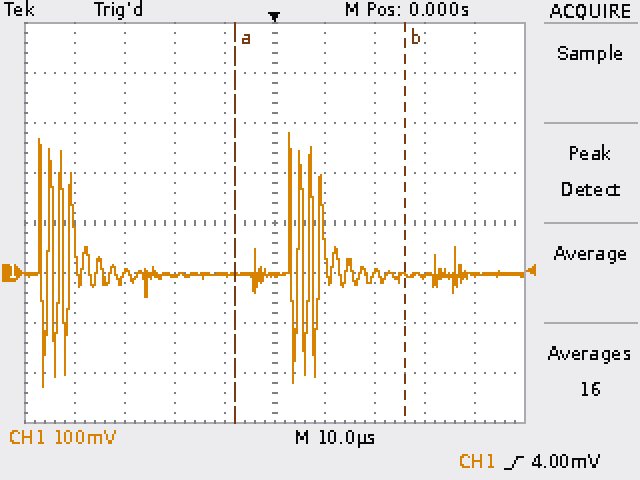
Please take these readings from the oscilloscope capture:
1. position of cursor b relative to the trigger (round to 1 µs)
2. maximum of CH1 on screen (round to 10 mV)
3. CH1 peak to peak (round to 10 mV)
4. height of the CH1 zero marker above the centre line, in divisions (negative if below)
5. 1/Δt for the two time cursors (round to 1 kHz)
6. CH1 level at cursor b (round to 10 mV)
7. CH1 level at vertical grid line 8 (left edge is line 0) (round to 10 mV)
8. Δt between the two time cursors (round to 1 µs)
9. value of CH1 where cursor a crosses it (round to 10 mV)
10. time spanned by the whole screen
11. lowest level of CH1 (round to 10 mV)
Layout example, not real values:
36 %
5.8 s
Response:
+26 µs
280 mV
510 mV
-1.0 div
29 kHz
-10 mV
-10 mV
34 µs
0 mV
100 µs
-230 mV
